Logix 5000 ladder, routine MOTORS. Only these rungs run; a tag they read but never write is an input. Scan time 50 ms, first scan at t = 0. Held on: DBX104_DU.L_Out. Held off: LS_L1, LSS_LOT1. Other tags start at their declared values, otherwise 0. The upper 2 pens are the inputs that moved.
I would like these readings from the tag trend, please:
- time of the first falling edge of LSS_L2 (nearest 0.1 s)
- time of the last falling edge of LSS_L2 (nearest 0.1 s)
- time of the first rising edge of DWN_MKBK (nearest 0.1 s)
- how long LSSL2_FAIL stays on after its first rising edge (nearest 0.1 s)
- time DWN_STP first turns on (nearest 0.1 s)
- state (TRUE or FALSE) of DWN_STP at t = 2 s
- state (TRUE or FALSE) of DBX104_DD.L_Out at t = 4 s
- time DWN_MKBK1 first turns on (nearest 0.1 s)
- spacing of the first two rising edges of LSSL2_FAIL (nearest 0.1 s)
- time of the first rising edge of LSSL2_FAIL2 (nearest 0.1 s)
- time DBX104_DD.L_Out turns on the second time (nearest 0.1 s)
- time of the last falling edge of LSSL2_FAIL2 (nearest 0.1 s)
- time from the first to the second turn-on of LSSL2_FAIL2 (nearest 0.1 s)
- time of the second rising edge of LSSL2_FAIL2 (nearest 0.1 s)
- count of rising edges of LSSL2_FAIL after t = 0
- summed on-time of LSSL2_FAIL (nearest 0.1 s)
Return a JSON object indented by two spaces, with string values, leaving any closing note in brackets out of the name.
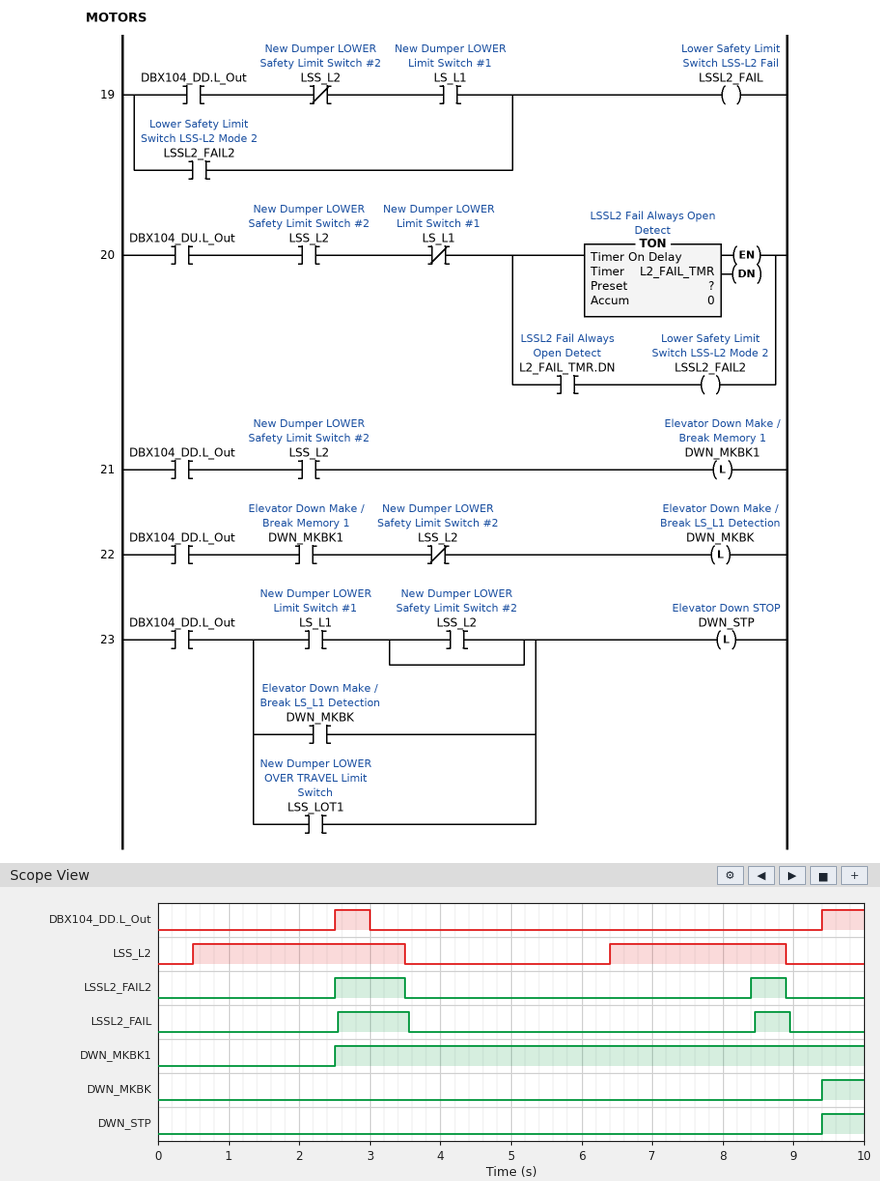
{
  "time of the first falling edge of LSS_L2": "3.5 s",
  "time of the last falling edge of LSS_L2": "8.9 s",
  "time of the first rising edge of DWN_MKBK": "9.4 s",
  "how long LSSL2_FAIL stays on after its first rising edge": "1.0 s",
  "time DWN_STP first turns on": "9.4 s",
  "state (TRUE or FALSE) of DWN_STP at t = 2 s": "FALSE",
  "state (TRUE or FALSE) of DBX104_DD.L_Out at t = 4 s": "FALSE",
  "time DWN_MKBK1 first turns on": "2.5 s",
  "spacing of the first two rising edges of LSSL2_FAIL": "5.9 s",
  "time of the first rising edge of LSSL2_FAIL2": "2.5 s",
  "time DBX104_DD.L_Out turns on the second time": "9.4 s",
  "time of the last falling edge of LSSL2_FAIL2": "8.9 s",
  "time from the first to the second turn-on of LSSL2_FAIL2": "5.9 s",
  "time of the second rising edge of LSSL2_FAIL2": "8.4 s",
  "count of rising edges of LSSL2_FAIL after t = 0": "2",
  "summed on-time of LSSL2_FAIL": "1.5 s"
}
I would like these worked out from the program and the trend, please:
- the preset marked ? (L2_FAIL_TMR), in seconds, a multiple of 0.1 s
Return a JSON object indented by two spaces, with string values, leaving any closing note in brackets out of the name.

{
  "the preset marked ? (L2_FAIL_TMR), in seconds, a multiple of 0.1 s": "2.0 s"
}
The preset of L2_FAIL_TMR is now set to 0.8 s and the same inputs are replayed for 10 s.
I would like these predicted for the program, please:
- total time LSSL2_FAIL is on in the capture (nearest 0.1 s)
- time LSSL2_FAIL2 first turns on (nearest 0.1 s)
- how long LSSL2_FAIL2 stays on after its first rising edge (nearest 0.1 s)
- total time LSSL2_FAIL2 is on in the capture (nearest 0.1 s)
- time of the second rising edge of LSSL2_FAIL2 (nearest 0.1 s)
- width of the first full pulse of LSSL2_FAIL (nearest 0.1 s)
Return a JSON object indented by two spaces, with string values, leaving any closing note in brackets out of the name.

{
  "total time LSSL2_FAIL is on in the capture": "3.9 s",
  "time LSSL2_FAIL2 first turns on": "1.3 s",
  "how long LSSL2_FAIL2 stays on after its first rising edge": "2.2 s",
  "total time LSSL2_FAIL2 is on in the capture": "3.9 s",
  "time of the second rising edge of LSSL2_FAIL2": "7.2 s",
  "width of the first full pulse of LSSL2_FAIL": "2.2 s"
}
